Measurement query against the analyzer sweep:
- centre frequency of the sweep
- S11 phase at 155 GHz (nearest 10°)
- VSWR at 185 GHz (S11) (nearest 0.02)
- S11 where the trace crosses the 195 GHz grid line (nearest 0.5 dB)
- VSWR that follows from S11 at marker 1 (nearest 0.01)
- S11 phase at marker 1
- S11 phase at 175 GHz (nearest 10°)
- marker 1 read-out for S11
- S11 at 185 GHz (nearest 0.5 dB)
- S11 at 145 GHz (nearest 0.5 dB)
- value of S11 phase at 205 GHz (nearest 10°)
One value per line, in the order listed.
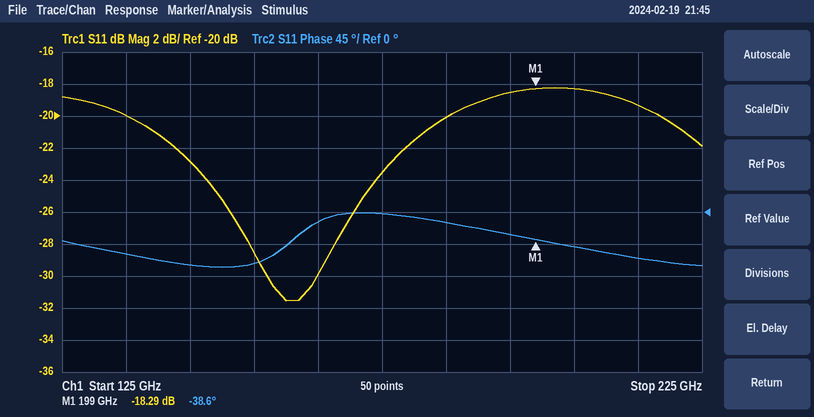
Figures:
175 GHz
-70°
1.22
-18.5 dB
1.28
-38.6°
0°
-18.29 dB
-20.0 dB
-23.0 dB
-50°
